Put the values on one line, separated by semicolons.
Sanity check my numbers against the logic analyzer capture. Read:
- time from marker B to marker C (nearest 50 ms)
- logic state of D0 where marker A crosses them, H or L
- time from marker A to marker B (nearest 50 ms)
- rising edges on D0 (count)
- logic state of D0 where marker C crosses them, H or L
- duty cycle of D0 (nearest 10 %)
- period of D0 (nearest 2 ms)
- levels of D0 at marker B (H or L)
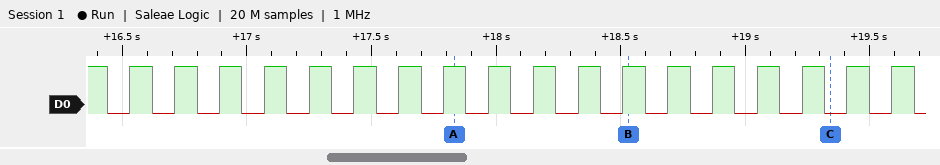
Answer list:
800 ms; D0=H; 700 ms; 18; D0=L; 50 %; 180 ms; D0=H
